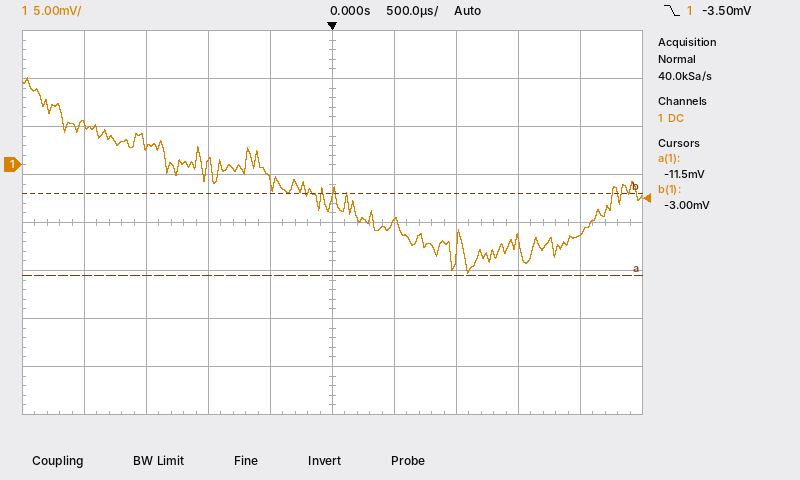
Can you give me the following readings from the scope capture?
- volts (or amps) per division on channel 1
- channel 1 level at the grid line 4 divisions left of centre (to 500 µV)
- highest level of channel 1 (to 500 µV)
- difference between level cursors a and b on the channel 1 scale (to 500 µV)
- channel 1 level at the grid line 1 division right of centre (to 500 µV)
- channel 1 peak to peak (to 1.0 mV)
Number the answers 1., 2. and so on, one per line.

1. 5 mV
2. 4.0 mV
3. 9.0 mV
4. 8.5 mV
5. -6.0 mV
6. 20.0 mV
